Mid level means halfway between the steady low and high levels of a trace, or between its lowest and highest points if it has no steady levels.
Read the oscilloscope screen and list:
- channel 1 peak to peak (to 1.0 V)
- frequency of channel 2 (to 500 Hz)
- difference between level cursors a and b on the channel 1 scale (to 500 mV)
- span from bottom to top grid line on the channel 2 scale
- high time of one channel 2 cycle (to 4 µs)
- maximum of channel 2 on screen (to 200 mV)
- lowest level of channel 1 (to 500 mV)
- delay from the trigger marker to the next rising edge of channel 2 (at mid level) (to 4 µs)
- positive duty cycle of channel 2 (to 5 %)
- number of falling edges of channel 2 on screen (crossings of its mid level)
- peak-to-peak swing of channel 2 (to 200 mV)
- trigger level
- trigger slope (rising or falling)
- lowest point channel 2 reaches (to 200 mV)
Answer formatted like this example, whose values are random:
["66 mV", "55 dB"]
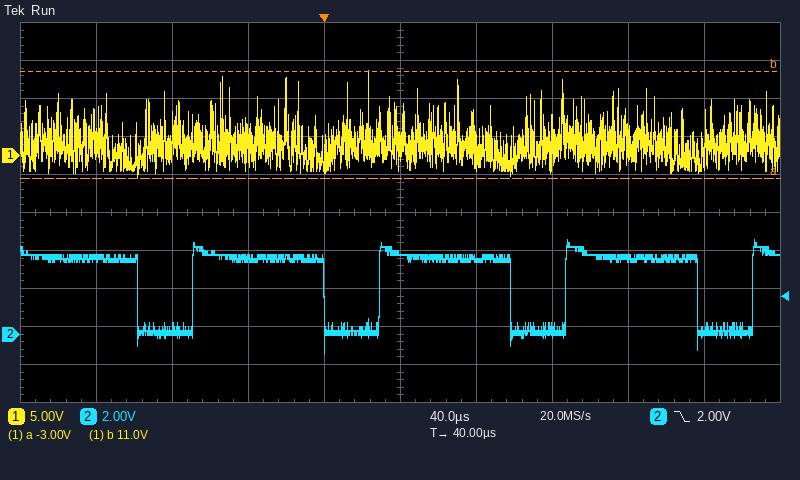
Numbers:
["14.0 V", "10.0 kHz", "14.0 V", "20 V", "68 µs", "5.0 V", "-3.0 V", "28 µs", "70 %", "4", "6.0 V", "2.00 V", "falling", "-1.0 V"]
